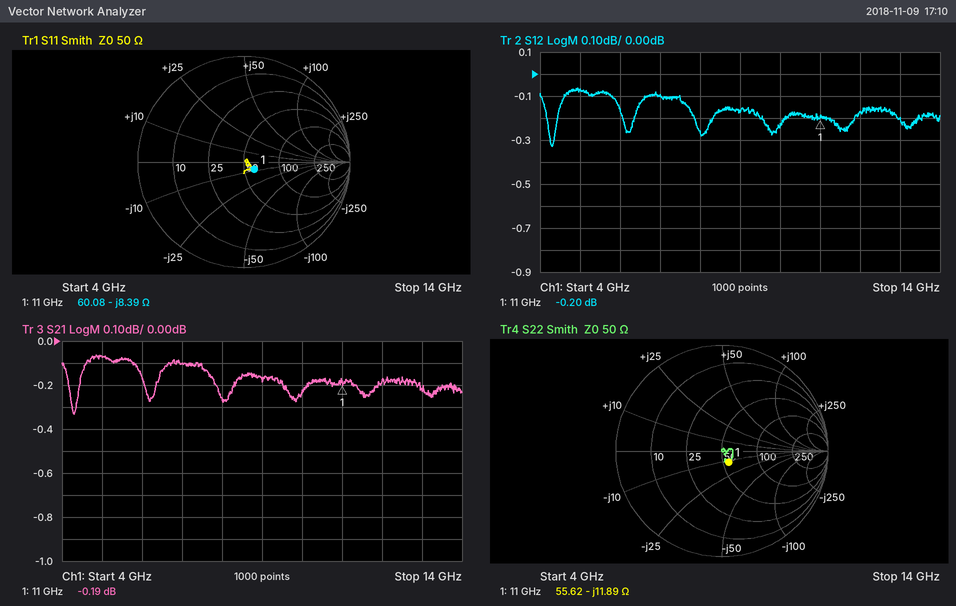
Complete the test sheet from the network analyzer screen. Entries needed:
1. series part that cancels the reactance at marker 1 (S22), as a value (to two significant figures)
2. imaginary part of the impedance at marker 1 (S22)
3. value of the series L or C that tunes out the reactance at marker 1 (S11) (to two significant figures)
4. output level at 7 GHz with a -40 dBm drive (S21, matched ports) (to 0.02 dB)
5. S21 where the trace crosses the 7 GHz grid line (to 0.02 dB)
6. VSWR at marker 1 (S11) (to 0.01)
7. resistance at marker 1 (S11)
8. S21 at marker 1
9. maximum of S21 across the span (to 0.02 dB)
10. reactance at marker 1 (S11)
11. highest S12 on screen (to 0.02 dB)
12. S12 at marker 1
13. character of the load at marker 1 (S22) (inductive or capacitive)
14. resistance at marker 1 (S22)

170 pH
-11.89 Ω
120 pH
-40.10 dBm
-0.10 dB
1.27
60.08 Ω
-0.19 dB
-0.06 dB
-8.39 Ω
-0.06 dB
-0.20 dB
capacitive
55.62 Ω
